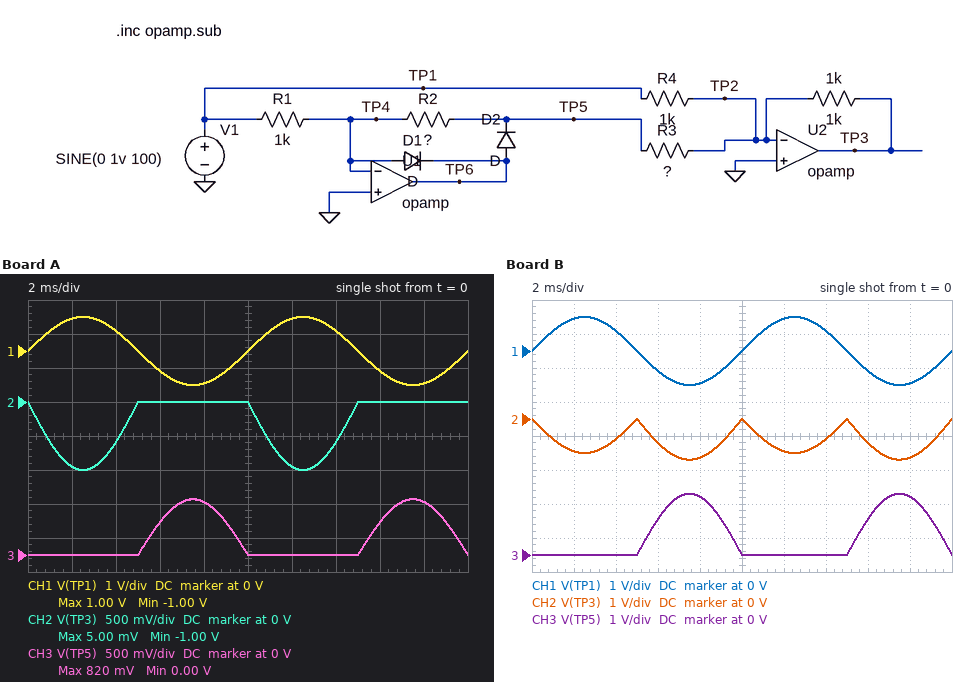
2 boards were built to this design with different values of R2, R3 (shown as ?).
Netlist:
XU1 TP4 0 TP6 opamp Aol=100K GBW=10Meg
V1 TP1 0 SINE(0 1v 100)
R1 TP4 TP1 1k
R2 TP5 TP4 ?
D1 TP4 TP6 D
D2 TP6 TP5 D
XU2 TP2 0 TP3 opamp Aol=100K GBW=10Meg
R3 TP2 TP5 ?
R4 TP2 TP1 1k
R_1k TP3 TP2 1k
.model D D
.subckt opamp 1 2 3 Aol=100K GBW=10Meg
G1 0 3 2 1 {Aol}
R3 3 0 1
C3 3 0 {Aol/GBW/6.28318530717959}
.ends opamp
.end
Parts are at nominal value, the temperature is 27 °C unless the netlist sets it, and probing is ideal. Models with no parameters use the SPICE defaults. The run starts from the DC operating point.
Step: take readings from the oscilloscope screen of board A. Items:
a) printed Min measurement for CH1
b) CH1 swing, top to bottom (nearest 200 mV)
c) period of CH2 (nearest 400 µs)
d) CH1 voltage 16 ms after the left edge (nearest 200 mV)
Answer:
-1.00 V
2.0 V
10.0 ms
-600 mV
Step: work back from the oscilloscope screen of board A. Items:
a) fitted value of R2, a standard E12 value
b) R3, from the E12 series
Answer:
820 Ω
820 Ω
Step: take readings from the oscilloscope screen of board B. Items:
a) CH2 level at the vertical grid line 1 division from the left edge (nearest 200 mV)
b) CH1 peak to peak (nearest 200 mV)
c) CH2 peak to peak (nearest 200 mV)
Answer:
-1.0 V
2.0 V
1.2 V
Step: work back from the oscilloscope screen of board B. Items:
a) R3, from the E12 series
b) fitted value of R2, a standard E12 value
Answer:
820 Ω
1.8 kΩ
